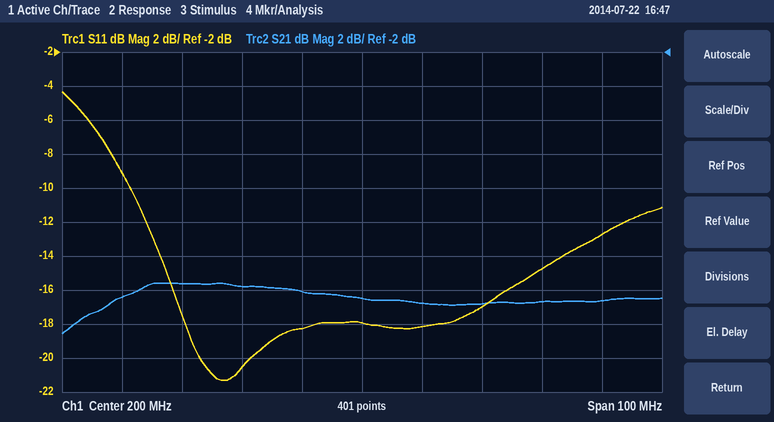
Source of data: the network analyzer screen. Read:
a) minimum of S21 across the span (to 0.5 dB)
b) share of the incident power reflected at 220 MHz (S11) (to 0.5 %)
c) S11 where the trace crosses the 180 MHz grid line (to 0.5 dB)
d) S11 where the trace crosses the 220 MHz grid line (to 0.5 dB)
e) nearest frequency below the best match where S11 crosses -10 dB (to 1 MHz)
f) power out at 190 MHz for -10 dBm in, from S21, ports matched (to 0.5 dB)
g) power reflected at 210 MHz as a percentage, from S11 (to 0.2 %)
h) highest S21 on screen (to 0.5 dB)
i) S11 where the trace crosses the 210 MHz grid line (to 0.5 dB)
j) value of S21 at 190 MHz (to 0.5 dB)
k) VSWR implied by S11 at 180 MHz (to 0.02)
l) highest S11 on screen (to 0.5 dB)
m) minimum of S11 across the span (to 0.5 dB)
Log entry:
-18.5 dB
2.0 %
-20.5 dB
-17.0 dB
161 MHz
-26.0 dBm
1.6 %
-15.5 dB
-18.0 dB
-16.0 dB
1.20
-4.5 dB
-21.5 dB
